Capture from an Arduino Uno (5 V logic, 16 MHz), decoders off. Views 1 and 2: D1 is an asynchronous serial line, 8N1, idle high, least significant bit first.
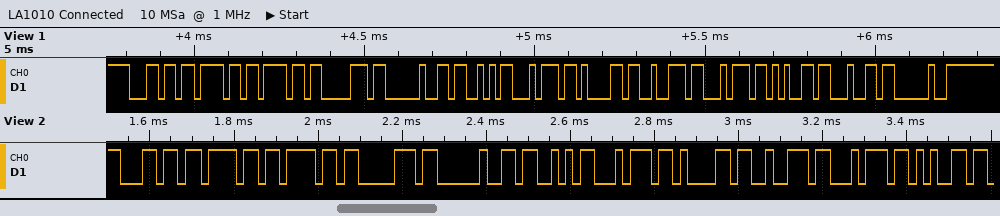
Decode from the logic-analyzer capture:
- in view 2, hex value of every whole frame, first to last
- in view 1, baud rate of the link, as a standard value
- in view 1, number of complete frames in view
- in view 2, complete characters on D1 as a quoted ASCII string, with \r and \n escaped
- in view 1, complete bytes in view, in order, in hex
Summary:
6C 6F 6F 70 20 53 74 61 72 74 65
57600 baud
13
"loop Starte"
0x6C 0x6F 0x6F 0x70 0x20 0x53 0x74 0x61 0x72 0x74 0x65 0x64 0x20
